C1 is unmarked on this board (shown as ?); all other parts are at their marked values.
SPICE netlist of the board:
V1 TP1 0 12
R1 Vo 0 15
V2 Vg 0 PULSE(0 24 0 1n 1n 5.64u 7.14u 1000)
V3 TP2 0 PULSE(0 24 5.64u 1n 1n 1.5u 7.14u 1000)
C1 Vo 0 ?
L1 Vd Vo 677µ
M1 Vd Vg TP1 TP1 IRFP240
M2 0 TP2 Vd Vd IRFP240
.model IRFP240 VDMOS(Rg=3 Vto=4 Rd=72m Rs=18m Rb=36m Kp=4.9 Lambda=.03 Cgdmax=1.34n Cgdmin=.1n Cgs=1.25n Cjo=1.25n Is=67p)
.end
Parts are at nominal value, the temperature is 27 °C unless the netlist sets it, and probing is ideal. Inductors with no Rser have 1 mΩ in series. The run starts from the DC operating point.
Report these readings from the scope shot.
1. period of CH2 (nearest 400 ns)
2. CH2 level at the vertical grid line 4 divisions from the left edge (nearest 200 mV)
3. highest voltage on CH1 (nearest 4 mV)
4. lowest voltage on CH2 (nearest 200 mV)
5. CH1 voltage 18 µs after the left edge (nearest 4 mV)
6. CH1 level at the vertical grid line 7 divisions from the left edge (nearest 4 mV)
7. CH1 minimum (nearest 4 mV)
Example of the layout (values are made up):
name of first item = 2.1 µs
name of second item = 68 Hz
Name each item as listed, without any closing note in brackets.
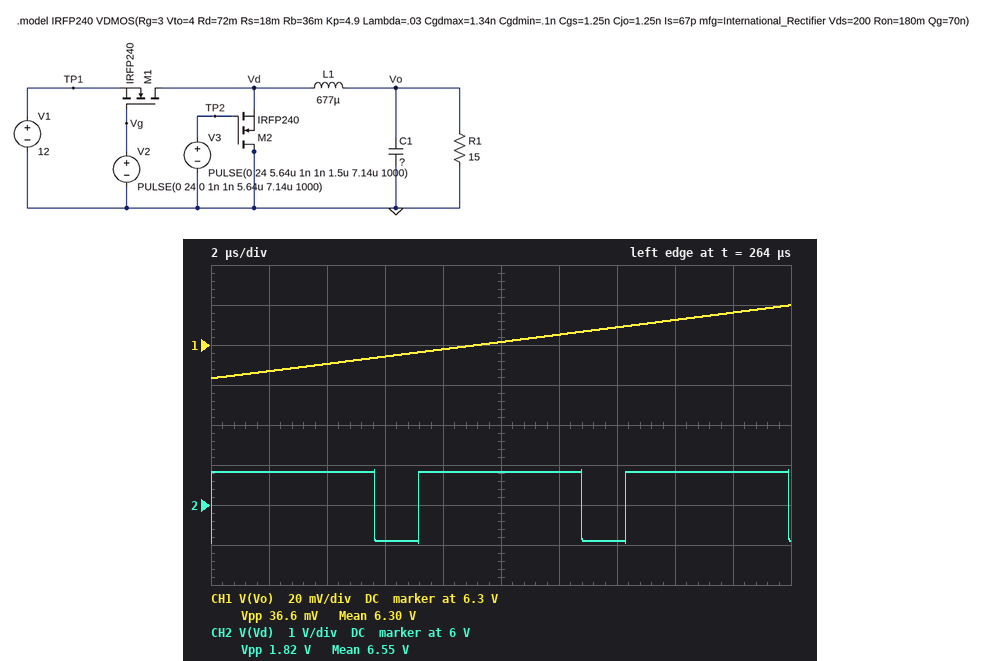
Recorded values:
period of CH2 = 7.2 µs
CH2 level at the vertical grid line 4 divisions from the left edge = 6.8 V
highest voltage on CH1 = 6.320 V
lowest voltage on CH2 = 5.0 V
CH1 voltage 18 µs after the left edge = 6.316 V
CH1 level at the vertical grid line 7 divisions from the left edge = 6.308 V
CH1 minimum = 6.284 V
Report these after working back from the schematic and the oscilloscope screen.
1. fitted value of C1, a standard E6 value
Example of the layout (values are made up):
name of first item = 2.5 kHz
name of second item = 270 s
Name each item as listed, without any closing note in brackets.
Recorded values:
fitted value of C1, a standard E6 value = 68 µF
